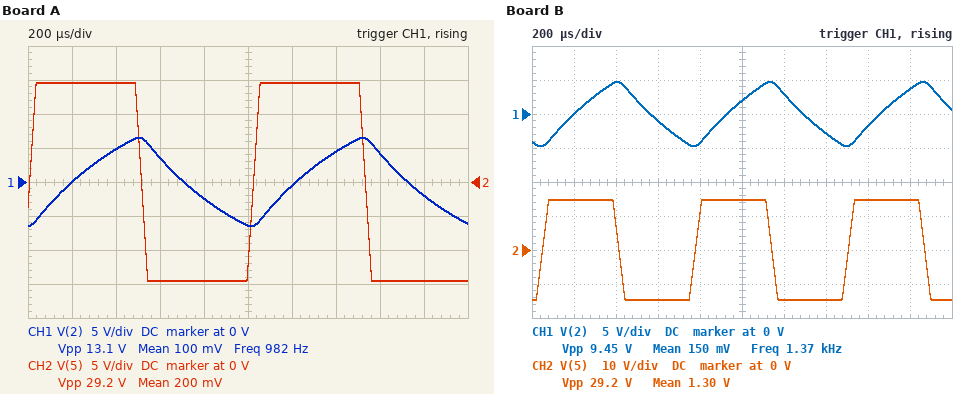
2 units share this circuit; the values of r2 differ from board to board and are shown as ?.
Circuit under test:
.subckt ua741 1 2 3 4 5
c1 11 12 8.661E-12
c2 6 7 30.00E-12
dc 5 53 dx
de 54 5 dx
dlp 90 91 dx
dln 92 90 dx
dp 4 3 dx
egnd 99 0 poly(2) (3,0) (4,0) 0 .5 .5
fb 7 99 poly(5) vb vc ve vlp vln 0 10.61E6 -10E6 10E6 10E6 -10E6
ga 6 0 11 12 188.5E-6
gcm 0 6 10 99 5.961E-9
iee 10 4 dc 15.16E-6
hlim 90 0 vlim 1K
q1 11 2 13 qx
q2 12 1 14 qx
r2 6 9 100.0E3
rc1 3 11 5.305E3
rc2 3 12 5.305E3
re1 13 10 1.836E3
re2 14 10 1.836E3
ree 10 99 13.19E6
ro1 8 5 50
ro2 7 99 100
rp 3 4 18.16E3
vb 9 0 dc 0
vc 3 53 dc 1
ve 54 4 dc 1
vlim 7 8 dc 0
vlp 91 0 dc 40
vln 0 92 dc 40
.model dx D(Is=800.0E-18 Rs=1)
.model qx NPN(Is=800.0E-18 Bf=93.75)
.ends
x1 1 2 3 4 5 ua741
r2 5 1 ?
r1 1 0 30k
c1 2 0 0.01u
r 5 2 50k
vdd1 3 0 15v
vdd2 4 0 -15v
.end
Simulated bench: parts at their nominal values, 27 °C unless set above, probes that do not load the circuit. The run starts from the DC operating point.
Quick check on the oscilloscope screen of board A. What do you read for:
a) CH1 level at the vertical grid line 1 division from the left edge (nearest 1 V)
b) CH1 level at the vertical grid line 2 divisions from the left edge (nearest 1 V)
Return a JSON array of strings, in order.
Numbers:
["0 V", "5 V"]
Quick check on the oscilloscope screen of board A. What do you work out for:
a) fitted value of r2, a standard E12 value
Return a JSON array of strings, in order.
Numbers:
["39 kΩ"]
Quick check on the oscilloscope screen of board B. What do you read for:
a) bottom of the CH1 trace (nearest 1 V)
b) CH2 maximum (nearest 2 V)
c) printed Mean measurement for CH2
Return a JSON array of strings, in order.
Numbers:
["-5 V", "14 V", "1.30 V"]
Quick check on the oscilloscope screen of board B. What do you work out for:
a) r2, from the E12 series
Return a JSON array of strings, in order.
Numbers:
["68 kΩ"]
